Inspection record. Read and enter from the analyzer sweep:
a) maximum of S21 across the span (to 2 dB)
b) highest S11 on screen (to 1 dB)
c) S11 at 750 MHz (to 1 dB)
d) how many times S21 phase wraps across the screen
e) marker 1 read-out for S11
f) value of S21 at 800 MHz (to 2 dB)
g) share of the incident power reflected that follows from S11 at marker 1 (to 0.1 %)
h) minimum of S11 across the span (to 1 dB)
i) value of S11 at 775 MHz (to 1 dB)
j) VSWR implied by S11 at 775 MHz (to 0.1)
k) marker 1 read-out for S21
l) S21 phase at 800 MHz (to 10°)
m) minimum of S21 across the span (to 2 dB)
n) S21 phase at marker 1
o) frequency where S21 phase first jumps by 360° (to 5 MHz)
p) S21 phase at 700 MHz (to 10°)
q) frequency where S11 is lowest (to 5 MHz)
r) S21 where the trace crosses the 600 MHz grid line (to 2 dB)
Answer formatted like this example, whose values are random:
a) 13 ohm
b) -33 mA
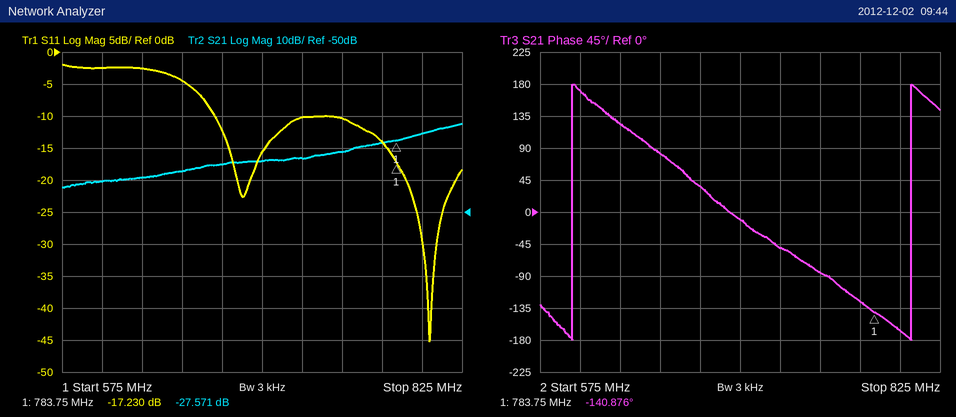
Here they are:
a) -22 dB
b) -2 dB
c) -10 dB
d) 2
e) -17.230 dB
f) -26 dB
g) 1.9 %
h) -45 dB
i) -14 dB
j) 1.5
k) -27.571 dB
l) -170°
m) -42 dB
n) -140.876°
o) 595 MHz
p) -10°
q) 805 MHz
r) -40 dB
